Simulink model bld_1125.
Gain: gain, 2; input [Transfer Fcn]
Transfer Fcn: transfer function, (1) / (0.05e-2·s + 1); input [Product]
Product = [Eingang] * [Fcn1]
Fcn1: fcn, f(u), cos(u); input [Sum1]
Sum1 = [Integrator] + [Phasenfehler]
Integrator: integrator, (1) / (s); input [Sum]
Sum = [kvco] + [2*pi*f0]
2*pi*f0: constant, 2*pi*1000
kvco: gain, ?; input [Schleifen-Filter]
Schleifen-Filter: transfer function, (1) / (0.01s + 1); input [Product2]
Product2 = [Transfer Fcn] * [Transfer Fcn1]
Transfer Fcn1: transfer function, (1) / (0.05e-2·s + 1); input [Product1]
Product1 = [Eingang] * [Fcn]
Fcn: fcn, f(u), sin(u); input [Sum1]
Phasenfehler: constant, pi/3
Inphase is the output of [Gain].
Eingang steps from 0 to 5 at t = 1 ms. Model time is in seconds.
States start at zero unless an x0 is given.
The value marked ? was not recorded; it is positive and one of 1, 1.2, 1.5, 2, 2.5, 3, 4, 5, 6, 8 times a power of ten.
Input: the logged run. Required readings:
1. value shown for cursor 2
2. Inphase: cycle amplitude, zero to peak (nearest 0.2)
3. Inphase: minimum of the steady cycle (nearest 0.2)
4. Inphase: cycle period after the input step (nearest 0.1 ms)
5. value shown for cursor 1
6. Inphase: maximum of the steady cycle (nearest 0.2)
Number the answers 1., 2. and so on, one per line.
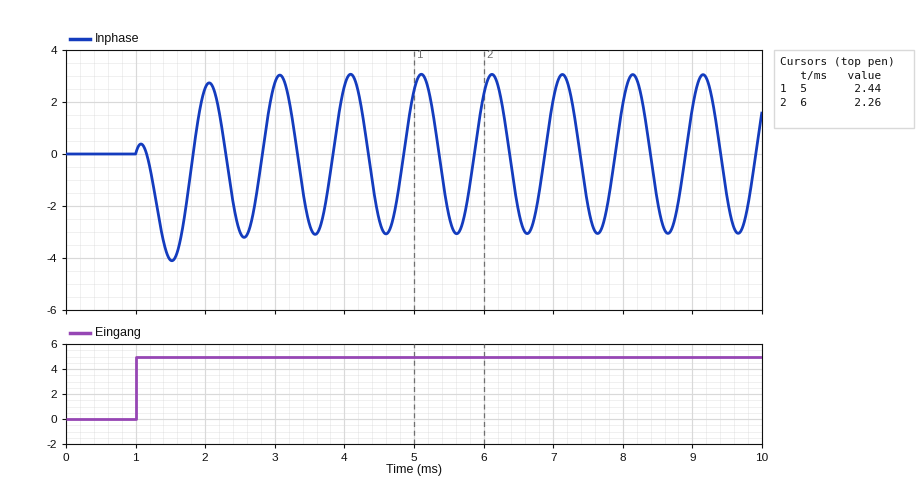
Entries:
1. 2.26
2. 3.0
3. -3.0
4. 1.0 ms
5. 2.44
6. 3.0
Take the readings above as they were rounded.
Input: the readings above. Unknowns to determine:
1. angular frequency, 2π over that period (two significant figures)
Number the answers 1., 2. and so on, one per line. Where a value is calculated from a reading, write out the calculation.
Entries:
1. 2π / 1 = 6.3 rad/ms
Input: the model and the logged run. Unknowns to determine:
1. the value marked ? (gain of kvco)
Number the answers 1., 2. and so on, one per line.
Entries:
1. 5000
